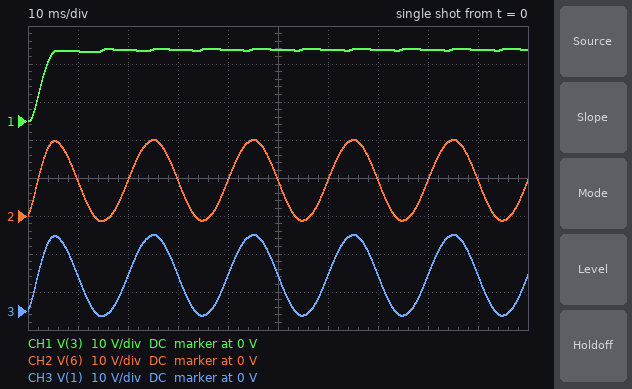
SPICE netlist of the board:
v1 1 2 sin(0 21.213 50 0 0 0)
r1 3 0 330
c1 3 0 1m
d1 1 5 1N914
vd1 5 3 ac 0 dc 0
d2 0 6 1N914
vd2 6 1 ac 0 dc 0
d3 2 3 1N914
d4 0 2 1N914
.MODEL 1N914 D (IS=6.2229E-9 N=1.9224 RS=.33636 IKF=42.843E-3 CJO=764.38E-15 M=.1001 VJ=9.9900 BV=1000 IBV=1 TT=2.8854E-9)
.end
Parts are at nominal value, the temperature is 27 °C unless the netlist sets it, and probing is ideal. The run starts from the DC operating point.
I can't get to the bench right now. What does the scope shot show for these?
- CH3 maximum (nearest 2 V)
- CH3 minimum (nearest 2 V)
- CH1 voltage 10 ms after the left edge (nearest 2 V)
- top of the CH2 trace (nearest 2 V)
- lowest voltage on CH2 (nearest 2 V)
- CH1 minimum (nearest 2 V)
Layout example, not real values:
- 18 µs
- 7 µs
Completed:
- 20 V
- -2 V
- 18 V
- 20 V
- -2 V
- 0 V
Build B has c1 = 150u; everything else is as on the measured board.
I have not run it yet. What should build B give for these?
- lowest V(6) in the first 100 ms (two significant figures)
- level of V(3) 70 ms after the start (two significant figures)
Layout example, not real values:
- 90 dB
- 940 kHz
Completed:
- -1.2 V
- 18 V
